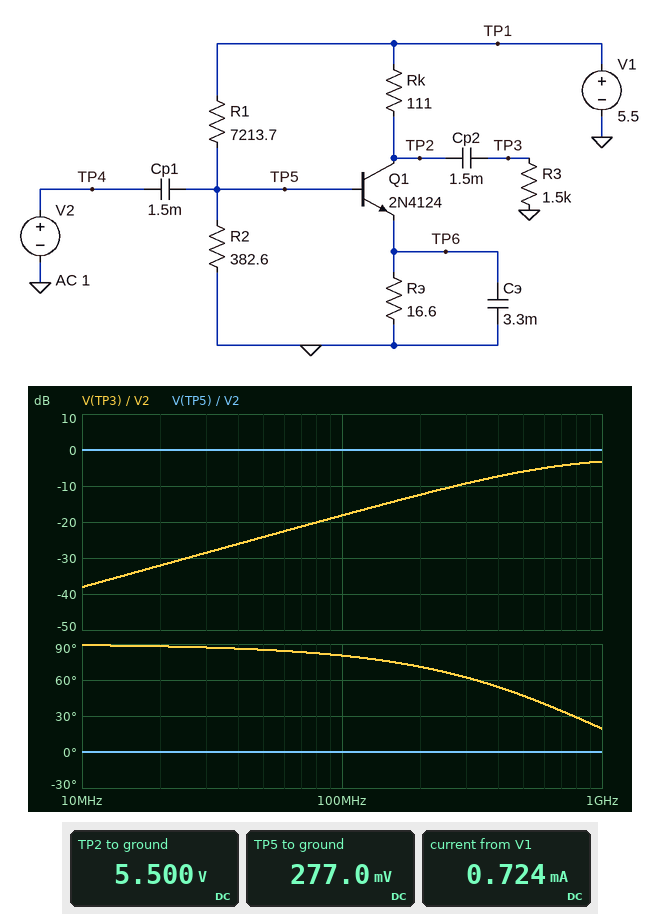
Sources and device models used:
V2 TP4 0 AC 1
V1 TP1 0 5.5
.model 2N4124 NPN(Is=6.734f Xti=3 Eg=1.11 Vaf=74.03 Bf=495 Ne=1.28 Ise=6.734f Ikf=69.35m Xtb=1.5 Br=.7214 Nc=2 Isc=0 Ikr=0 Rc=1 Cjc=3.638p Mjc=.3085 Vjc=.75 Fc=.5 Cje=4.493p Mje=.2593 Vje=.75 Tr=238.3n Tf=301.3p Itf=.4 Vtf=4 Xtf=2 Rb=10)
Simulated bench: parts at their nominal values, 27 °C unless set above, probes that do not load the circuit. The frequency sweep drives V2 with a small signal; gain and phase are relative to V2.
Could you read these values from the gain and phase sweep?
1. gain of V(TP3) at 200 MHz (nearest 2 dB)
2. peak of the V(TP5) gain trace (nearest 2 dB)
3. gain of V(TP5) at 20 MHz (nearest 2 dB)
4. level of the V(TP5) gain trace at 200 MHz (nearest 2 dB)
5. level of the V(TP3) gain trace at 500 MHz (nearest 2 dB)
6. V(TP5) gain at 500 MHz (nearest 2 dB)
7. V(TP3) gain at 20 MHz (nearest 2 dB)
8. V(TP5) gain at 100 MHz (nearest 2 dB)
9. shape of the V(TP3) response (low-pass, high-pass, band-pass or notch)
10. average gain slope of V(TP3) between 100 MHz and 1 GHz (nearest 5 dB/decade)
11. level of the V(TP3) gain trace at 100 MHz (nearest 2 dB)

-12 dB
0 dB
0 dB
0 dB
-6 dB
0 dB
-32 dB
0 dB
high-pass
15 dB/decade
-18 dB
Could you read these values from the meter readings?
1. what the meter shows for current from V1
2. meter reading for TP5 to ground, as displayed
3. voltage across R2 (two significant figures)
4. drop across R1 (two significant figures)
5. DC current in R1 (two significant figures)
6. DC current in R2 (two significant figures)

0.724 mA
277.0 mV
280 mV
5.2 V
720 µA
720 µA
